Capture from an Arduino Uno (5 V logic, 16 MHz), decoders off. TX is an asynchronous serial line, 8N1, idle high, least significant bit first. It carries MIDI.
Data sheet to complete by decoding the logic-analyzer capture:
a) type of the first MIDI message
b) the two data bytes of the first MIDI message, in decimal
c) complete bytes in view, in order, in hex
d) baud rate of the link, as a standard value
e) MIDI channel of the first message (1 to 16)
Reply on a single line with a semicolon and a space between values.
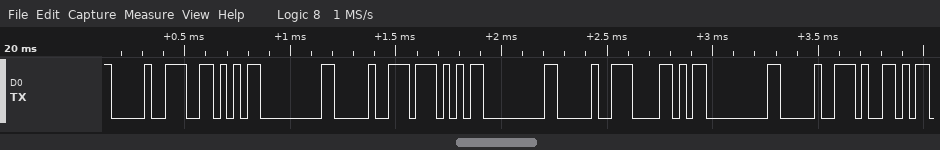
Note On; 86, 0; 90 56 00 90 57 00 90 58 00 90 59; 31250 baud; 1
